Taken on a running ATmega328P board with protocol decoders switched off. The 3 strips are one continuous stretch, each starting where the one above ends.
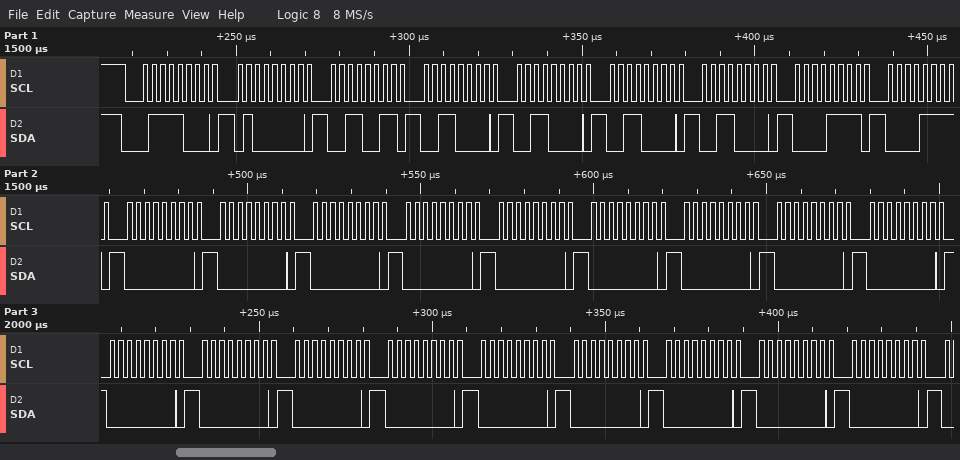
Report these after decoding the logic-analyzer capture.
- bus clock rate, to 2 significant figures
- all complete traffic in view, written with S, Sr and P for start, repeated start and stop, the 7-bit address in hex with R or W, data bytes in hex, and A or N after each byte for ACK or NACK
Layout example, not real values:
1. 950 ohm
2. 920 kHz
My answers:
1. 400 kHz
2. S 3CW A 40 A 33 A 30 A 30 A 30 A 30 A 0F A 0F A 00 A 00 A 00 A 00 A 00 A 00 A 00 A 00 A 00 A 00 A 00 A 00 A 00 A 00 A 00 A 00 A 00 A 00 A
